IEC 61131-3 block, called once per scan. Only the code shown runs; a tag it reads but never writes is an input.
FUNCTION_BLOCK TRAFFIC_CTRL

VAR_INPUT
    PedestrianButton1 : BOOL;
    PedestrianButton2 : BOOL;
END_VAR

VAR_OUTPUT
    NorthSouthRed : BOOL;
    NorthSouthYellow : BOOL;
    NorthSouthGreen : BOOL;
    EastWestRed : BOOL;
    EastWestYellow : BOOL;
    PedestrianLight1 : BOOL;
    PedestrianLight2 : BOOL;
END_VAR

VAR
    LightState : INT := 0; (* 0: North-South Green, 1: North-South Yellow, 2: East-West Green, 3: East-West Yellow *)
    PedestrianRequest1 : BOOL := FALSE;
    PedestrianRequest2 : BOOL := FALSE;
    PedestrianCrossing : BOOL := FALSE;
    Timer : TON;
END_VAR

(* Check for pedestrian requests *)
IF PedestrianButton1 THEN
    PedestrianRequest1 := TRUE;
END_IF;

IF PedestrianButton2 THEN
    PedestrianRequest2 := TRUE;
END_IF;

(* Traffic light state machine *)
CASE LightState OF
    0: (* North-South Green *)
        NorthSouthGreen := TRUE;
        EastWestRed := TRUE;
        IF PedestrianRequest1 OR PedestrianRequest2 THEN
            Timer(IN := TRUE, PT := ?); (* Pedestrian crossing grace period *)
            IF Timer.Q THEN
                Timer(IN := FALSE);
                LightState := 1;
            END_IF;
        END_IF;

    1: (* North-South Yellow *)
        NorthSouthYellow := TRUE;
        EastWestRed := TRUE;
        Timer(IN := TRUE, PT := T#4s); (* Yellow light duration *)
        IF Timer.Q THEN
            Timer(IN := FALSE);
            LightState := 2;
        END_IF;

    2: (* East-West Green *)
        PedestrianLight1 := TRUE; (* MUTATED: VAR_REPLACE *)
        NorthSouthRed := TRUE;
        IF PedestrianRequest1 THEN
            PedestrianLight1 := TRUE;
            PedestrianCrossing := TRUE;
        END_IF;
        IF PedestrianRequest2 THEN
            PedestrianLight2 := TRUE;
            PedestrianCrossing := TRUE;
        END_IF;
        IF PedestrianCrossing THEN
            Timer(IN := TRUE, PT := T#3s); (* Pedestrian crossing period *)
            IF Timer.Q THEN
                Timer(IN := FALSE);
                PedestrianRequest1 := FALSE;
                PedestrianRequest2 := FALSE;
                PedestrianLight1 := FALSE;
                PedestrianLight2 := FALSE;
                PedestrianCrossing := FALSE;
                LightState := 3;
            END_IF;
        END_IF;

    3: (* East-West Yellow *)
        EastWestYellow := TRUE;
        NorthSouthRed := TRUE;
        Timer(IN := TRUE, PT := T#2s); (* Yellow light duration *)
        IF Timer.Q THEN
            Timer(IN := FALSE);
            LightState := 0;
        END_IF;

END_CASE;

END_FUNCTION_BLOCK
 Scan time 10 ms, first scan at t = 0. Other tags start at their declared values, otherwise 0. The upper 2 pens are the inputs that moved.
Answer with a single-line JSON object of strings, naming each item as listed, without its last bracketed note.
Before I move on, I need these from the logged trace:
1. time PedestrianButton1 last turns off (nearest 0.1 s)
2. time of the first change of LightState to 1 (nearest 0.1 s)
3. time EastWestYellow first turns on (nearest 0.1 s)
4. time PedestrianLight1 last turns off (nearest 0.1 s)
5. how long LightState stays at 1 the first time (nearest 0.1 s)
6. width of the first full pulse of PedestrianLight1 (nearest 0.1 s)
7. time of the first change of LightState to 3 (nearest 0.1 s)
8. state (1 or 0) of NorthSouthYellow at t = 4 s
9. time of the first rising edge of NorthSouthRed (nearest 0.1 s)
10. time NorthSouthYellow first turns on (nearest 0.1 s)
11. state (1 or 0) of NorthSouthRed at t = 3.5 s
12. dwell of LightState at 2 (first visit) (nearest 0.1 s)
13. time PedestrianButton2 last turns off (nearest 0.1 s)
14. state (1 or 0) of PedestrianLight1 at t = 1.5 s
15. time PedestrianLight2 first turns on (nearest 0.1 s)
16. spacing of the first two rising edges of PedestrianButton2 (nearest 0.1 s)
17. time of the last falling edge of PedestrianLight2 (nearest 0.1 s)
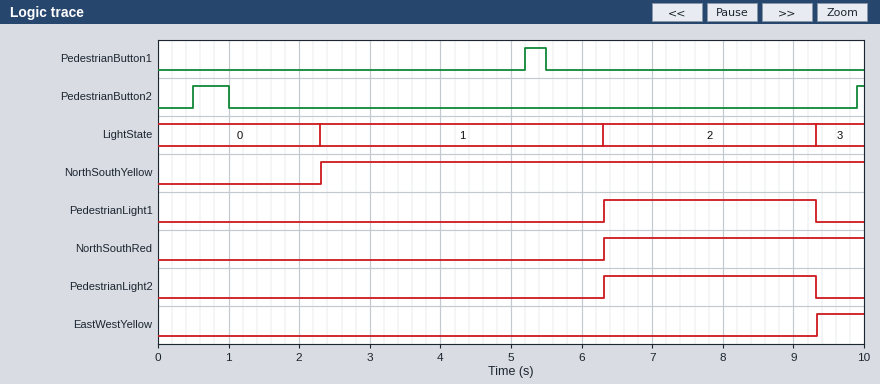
{"time PedestrianButton1 last turns off": "5.5 s", "time of the first change of LightState to 1": "2.3 s", "time EastWestYellow first turns on": "9.3 s", "time PedestrianLight1 last turns off": "9.3 s", "how long LightState stays at 1 the first time": "4.0 s", "width of the first full pulse of PedestrianLight1": "3.0 s", "time of the first change of LightState to 3": "9.3 s", "state (1 or 0) of NorthSouthYellow at t = 4 s": "1", "time of the first rising edge of NorthSouthRed": "6.3 s", "time NorthSouthYellow first turns on": "2.3 s", "state (1 or 0) of NorthSouthRed at t = 3.5 s": "0", "dwell of LightState at 2 (first visit)": "3.0 s", "time PedestrianButton2 last turns off": "1.0 s", "state (1 or 0) of PedestrianLight1 at t = 1.5 s": "0", "time PedestrianLight2 first turns on": "6.3 s", "spacing of the first two rising edges of PedestrianButton2": "9.4 s", "time of the last falling edge of PedestrianLight2": "9.3 s"}
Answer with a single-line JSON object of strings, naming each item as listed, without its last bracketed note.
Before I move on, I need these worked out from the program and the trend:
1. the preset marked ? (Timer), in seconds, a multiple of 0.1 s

{"the preset marked ? (Timer), in seconds, a multiple of 0.1 s": "1.8 s"}
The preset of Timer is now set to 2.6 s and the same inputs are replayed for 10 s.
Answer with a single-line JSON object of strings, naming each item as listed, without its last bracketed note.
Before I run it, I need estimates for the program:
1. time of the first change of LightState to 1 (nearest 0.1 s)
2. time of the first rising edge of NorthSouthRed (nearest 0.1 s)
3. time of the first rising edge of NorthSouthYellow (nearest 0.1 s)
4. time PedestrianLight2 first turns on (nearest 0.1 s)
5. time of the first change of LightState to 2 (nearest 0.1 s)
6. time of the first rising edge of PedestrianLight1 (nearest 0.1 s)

{"time of the first change of LightState to 1": "3.1 s", "time of the first rising edge of NorthSouthRed": "7.1 s", "time of the first rising edge of NorthSouthYellow": "3.1 s", "time PedestrianLight2 first turns on": "7.1 s", "time of the first change of LightState to 2": "7.1 s", "time of the first rising edge of PedestrianLight1": "7.1 s"}
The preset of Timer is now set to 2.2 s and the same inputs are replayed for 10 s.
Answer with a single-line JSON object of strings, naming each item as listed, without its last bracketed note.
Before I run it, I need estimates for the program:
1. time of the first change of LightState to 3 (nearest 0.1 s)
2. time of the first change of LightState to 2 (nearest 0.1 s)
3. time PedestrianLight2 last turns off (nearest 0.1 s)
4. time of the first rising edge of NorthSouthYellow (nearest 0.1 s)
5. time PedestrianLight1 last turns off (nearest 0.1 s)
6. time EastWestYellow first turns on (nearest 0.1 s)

{"time of the first change of LightState to 3": "9.7 s", "time of the first change of LightState to 2": "6.7 s", "time PedestrianLight2 last turns off": "9.7 s", "time of the first rising edge of NorthSouthYellow": "2.7 s", "time PedestrianLight1 last turns off": "9.7 s", "time EastWestYellow first turns on": "9.7 s"}
